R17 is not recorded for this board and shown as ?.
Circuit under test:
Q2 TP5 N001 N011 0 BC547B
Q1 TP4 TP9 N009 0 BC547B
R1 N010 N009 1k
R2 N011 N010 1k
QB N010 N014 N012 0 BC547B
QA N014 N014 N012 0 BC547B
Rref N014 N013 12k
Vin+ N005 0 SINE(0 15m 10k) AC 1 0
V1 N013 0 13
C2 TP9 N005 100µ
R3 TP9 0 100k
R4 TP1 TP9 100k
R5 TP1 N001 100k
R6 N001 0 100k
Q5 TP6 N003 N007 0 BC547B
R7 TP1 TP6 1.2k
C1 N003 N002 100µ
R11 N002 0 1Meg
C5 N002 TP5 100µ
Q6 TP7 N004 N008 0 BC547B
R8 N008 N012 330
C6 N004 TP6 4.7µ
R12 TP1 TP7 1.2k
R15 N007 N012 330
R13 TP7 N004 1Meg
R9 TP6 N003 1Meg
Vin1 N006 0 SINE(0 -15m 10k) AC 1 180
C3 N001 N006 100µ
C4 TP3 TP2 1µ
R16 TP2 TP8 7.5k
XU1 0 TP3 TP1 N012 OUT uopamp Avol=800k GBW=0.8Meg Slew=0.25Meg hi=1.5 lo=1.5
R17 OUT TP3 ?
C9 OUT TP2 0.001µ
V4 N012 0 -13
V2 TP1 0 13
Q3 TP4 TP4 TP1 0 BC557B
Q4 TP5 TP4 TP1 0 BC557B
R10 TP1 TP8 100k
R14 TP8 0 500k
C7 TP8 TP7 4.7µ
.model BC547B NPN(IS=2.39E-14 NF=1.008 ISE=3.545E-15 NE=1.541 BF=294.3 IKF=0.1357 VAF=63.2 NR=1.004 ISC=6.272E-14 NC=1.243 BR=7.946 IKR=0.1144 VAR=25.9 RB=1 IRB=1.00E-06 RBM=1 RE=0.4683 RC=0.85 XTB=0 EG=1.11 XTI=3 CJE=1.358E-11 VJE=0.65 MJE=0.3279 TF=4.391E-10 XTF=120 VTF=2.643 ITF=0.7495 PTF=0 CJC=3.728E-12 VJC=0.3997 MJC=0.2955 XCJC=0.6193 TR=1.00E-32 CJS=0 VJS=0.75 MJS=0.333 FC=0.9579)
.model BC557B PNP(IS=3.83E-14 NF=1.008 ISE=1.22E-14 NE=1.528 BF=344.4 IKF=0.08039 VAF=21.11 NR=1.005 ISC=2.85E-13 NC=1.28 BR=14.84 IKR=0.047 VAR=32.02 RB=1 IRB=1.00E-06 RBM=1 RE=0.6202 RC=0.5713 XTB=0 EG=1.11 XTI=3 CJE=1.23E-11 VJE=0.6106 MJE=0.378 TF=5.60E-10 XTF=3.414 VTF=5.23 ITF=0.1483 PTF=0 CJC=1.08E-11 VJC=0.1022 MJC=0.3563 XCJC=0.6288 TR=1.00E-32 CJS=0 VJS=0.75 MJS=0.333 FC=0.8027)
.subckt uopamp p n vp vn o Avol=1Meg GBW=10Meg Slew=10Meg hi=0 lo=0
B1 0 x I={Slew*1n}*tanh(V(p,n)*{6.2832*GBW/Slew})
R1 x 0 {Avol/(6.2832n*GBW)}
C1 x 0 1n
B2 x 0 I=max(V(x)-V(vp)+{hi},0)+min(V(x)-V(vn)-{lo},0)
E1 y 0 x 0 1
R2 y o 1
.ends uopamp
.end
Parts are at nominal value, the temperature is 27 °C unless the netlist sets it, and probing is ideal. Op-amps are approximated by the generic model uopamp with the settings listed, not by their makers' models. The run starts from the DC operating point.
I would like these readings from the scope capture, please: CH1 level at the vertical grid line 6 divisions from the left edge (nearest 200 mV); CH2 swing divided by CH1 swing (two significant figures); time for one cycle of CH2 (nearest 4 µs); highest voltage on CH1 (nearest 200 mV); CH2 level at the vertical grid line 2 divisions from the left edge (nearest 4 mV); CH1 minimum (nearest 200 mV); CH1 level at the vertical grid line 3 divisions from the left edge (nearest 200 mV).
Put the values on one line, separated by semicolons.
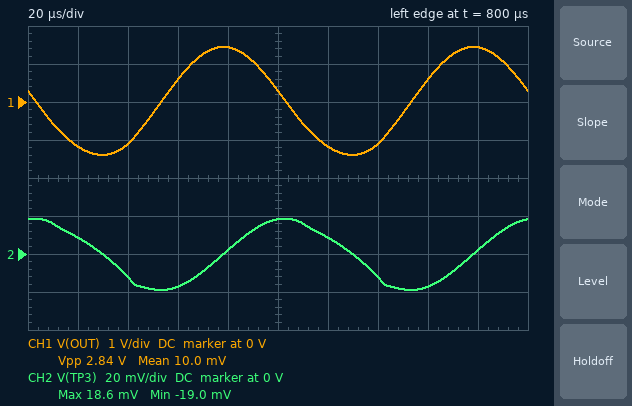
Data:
-1.2 V; 0.013; 100 µs; 1.4 V; -12 mV; -1.4 V; 600 mV
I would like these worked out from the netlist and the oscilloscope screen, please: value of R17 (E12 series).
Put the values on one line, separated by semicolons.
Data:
2.7 kΩ
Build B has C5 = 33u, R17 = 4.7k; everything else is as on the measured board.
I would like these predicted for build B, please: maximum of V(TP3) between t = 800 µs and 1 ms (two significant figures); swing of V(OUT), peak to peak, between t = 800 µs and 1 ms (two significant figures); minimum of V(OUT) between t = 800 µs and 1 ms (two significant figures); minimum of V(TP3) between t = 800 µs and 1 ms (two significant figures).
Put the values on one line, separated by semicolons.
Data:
35 mV; 4.8 V; -2.4 V; -36 mV
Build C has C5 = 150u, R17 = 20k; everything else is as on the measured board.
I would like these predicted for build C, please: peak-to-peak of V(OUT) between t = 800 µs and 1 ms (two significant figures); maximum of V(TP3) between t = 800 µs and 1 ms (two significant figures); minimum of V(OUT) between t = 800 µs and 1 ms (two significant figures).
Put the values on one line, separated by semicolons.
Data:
11 V; 1.2 V; -5.4 V
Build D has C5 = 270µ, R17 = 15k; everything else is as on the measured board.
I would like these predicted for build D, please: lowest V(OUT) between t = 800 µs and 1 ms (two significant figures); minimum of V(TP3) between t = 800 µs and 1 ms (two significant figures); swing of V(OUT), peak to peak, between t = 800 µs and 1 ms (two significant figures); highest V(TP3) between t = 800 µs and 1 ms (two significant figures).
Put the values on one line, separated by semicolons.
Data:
-5.2 V; -1.0 V; 10 V; 830 mV
